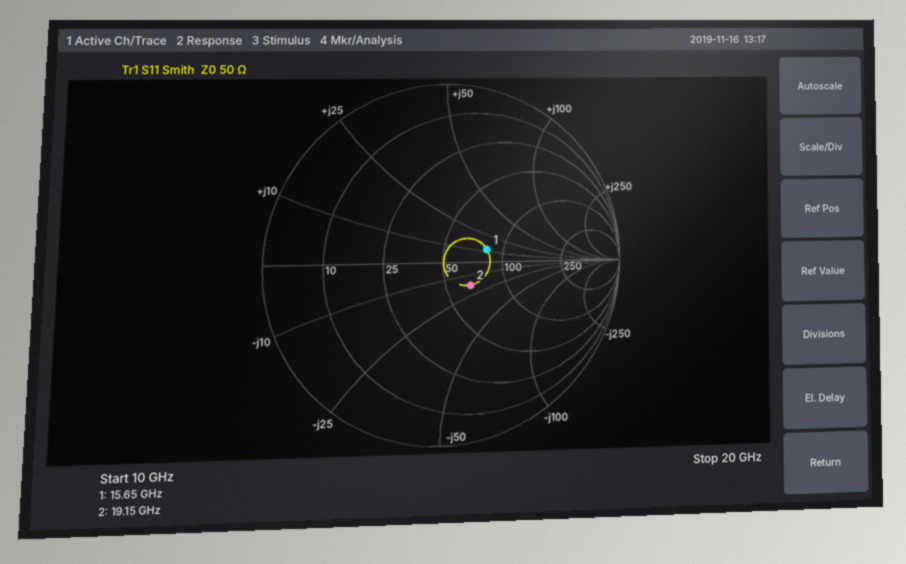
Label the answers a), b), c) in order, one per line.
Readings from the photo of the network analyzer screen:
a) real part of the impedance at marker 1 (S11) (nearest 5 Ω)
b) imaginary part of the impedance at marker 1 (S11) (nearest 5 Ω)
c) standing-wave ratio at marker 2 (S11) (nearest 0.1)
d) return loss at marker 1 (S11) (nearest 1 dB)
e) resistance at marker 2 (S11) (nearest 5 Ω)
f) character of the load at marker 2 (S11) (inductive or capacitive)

a) 80 Ω
b) +10 Ω
c) 1.5
d) 12 dB
e) 65 Ω
f) capacitive
